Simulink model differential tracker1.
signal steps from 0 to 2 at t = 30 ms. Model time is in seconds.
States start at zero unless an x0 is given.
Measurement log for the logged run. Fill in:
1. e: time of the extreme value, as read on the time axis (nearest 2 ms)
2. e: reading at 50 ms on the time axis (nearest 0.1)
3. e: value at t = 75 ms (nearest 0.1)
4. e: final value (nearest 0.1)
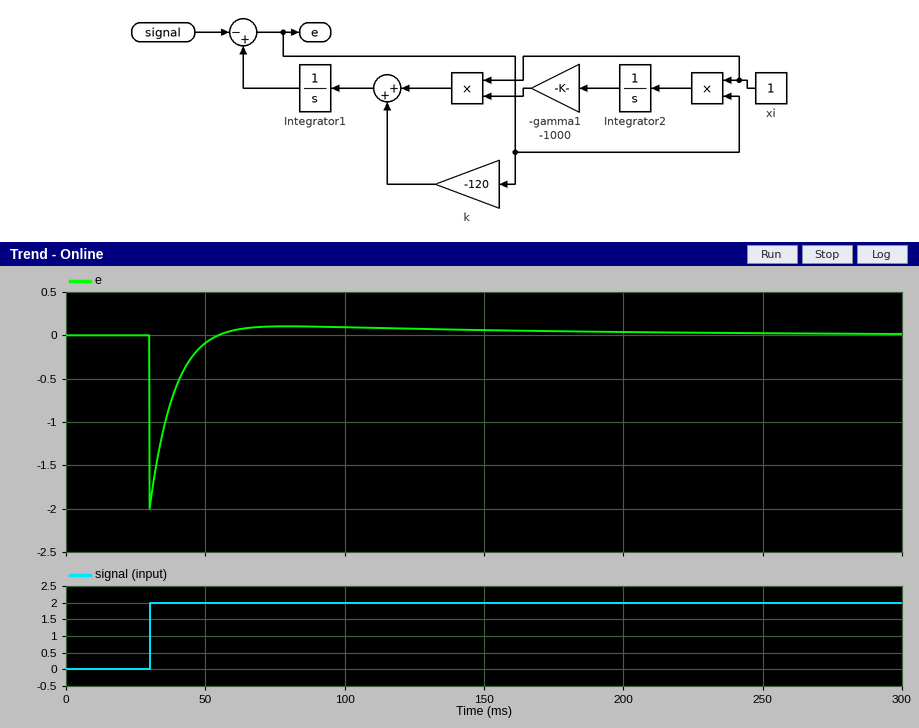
30 ms
-0.1
0.1
0.0
